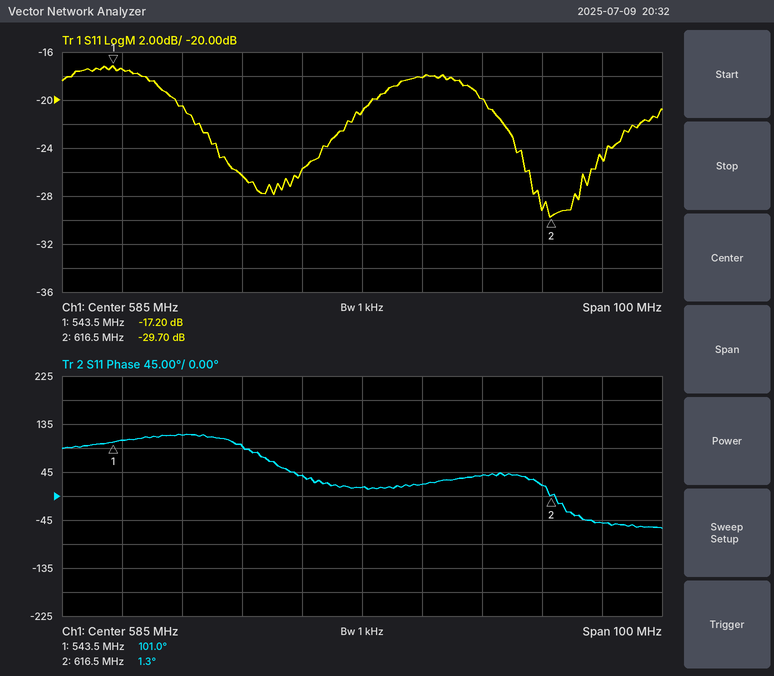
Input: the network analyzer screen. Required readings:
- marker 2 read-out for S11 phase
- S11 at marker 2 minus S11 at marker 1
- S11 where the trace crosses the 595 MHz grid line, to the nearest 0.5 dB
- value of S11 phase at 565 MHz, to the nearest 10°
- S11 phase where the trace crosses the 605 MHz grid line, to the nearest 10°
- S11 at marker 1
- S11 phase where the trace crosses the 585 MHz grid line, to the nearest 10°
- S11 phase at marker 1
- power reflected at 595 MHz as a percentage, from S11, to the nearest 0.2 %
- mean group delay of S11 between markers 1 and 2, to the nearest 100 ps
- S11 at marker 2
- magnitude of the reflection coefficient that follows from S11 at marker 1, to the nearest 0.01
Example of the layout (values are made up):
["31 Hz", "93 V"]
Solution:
["1.3°", "-12.50 dB", "-18.0 dB", "90°", "40°", "-17.20 dB", "20°", "101.0°", "1.6 %", "3.8 ns", "-29.70 dB", "0.14"]
